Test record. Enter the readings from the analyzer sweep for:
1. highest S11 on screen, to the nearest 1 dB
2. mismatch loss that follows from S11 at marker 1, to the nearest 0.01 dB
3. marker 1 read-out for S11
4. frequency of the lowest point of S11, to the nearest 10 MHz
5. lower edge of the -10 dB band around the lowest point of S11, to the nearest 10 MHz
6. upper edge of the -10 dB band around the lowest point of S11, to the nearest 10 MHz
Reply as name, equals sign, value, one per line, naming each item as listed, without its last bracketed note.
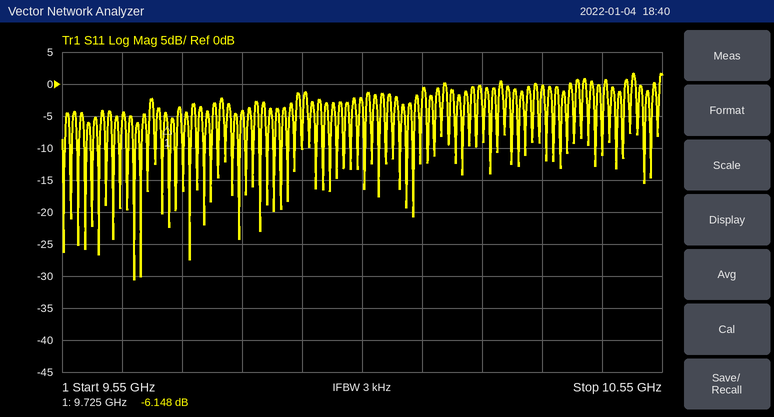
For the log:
highest S11 on screen, to the nearest 1 dB = 2 dB
mismatch loss that follows from S11 at marker 1, to the nearest 0.01 dB = 1.21 dB
marker 1 read-out for S11 = -6.148 dB
frequency of the lowest point of S11, to the nearest 10 MHz = 9.67 GHz
lower edge of the -10 dB band around the lowest point of S11, to the nearest 10 MHz = 9.67 GHz
upper edge of the -10 dB band around the lowest point of S11, to the nearest 10 MHz = 9.67 GHz
